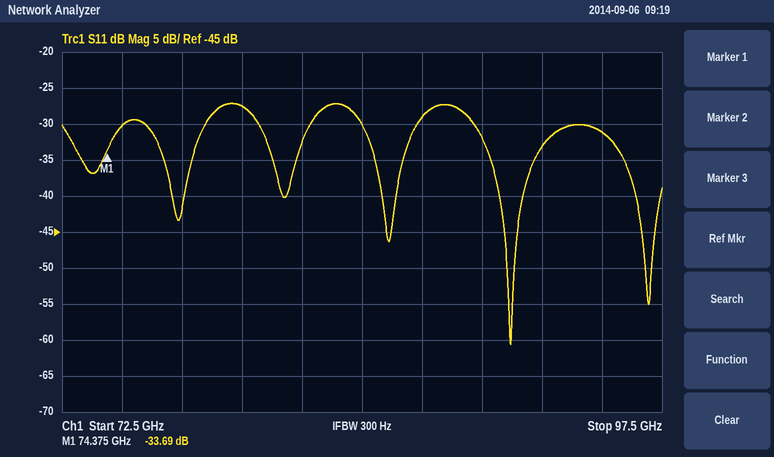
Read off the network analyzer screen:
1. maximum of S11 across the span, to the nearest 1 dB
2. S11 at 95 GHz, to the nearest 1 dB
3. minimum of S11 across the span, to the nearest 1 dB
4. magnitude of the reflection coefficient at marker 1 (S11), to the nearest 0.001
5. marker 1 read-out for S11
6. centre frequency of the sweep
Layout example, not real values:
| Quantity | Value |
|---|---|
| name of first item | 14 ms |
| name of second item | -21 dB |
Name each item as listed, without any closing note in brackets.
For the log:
| Quantity | Value |
|---|---|
| maximum of S11 across the span, to the nearest 1 dB | -27 dB |
| S11 at 95 GHz, to the nearest 1 dB | -31 dB |
| minimum of S11 across the span, to the nearest 1 dB | -61 dB |
| magnitude of the reflection coefficient at marker 1 (S11), to the nearest 0.001 | 0.021 |
| marker 1 read-out for S11 | -33.69 dB |
| centre frequency of the sweep | 85 GHz |
